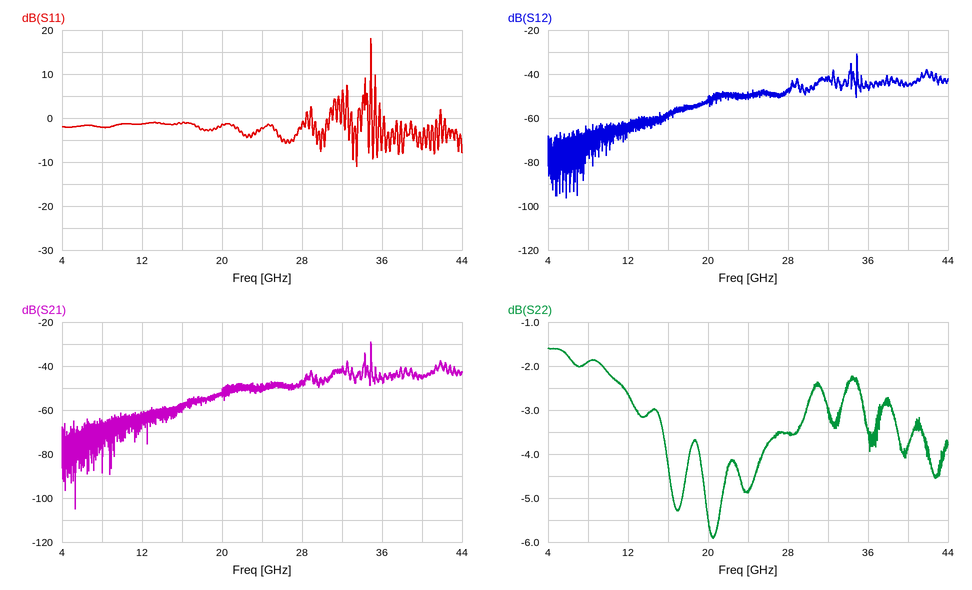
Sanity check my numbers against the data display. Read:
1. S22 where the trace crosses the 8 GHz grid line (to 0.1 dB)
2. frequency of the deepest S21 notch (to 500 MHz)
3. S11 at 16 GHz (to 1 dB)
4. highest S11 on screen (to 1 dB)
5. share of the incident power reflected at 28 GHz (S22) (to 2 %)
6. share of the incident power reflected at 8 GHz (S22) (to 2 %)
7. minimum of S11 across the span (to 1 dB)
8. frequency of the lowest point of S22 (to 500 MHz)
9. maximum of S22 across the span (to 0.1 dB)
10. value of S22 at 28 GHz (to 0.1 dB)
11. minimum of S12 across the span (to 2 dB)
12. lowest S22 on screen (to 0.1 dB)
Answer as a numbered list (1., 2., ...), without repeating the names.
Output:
1. -1.9 dB
2. 5.5 GHz
3. -1 dB
4. 18 dB
5. 44 %
6. 64 %
7. -11 dB
8. 20.5 GHz
9. -1.6 dB
10. -3.5 dB
11. -96 dB
12. -5.9 dB
